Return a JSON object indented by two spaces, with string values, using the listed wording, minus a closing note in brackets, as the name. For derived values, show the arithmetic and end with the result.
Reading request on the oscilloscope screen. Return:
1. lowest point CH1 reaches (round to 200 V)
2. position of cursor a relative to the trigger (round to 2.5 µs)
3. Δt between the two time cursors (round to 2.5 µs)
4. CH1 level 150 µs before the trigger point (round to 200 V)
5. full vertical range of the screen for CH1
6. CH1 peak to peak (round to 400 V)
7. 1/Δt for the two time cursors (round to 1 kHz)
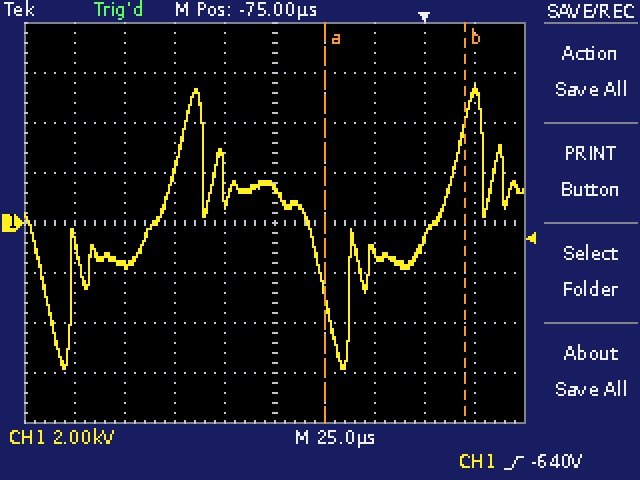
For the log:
{
  "lowest point CH1 reaches": "-5.8 kV",
  "position of cursor a relative to the trigger": "-50.0 µs",
  "Δt between the two time cursors": "70.0 µs",
  "CH1 level 150 µs before the trigger point": "-1.6 kV",
  "full vertical range of the screen for CH1": "16 kV",
  "CH1 peak to peak": "11.2 kV",
  "1/Δt for the two time cursors": "1 / 70.0 µs ≈ 14 kHz"
}
